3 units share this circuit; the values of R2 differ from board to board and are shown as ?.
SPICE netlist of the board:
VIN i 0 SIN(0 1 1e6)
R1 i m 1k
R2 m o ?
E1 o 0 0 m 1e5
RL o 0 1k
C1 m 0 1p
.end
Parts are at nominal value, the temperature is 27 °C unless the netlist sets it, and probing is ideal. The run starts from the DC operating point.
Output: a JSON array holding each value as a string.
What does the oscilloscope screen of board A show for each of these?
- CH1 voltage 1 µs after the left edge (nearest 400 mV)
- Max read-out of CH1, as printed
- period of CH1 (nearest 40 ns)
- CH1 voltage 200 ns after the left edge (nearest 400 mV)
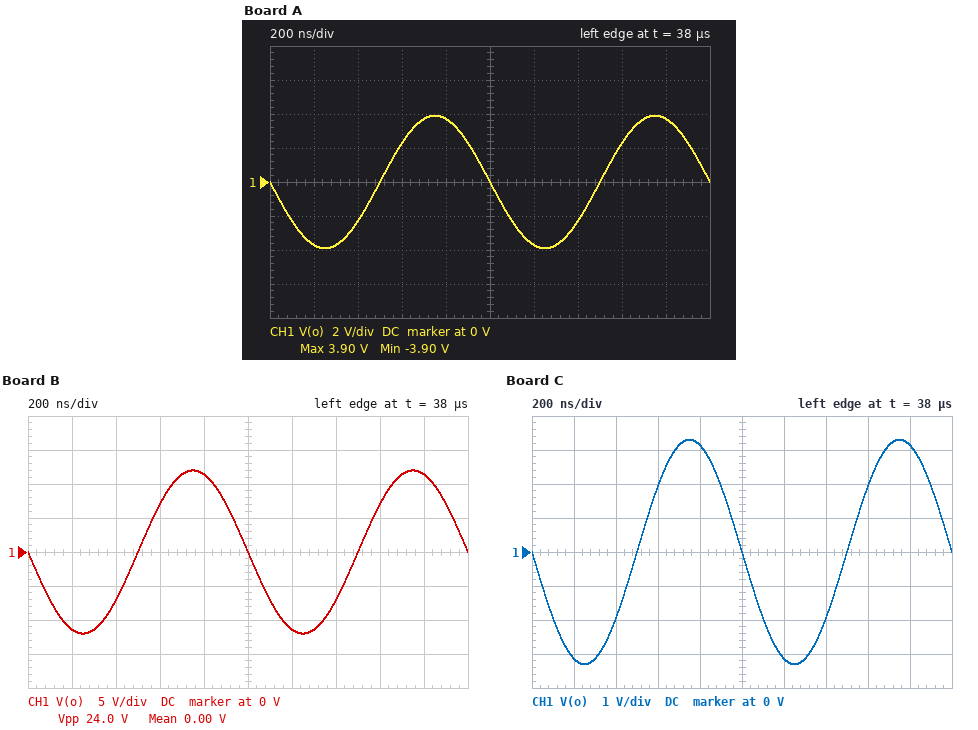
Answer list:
["0 V", "3.90 V", "1.00 µs", "-3.6 V"]
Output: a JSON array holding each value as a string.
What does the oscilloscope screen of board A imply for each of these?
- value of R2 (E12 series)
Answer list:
["3.9 kΩ"]
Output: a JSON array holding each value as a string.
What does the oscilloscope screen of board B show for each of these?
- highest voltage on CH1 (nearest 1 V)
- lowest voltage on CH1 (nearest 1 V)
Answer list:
["12 V", "-12 V"]
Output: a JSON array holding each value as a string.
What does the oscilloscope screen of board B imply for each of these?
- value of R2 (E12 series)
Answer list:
["12 kΩ"]
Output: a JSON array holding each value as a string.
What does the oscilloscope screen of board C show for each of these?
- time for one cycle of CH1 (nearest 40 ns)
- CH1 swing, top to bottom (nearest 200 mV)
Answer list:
["1.00 µs", "6.6 V"]
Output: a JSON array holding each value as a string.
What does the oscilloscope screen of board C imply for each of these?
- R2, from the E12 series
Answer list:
["3.3 kΩ"]
